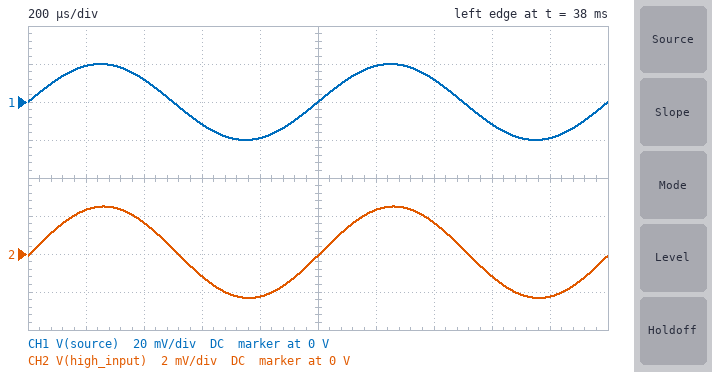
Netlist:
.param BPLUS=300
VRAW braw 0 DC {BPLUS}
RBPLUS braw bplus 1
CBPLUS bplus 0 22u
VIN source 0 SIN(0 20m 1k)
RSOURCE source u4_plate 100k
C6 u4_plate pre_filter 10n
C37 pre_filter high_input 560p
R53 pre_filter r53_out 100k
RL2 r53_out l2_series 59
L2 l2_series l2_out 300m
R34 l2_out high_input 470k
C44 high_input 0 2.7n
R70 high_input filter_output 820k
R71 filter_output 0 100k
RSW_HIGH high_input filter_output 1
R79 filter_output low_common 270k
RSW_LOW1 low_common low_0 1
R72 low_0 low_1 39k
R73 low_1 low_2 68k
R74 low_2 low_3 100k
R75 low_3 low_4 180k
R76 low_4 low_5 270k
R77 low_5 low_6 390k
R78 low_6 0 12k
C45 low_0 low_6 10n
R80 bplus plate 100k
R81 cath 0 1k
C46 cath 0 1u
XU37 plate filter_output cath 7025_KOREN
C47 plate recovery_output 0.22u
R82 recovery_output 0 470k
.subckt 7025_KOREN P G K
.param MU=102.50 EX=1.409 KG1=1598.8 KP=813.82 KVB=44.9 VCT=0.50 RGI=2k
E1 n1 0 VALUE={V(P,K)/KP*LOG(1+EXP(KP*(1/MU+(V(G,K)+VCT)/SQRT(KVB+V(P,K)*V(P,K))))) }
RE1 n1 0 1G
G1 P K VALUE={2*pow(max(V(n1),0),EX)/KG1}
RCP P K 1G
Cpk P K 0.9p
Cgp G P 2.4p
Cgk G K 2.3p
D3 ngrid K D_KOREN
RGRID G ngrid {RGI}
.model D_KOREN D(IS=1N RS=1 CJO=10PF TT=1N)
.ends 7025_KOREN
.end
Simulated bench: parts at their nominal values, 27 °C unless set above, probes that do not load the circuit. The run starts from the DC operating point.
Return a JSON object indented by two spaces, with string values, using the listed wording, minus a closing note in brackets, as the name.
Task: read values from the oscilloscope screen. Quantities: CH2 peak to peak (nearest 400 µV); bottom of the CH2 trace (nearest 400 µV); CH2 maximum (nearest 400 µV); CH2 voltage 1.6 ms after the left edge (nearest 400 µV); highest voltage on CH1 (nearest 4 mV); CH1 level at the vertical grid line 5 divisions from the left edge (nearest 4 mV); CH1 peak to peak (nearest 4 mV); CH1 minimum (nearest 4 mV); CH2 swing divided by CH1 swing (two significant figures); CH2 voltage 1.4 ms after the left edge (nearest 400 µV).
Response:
{
  "CH2 peak to peak": "4.8 mV",
  "bottom of the CH2 trace": "-2.4 mV",
  "CH2 maximum": "2.4 mV",
  "CH2 voltage 1.6 ms after the left edge": "-1.2 mV",
  "highest voltage on CH1": "20 mV",
  "CH1 level at the vertical grid line 5 divisions from the left edge": "0 V",
  "CH1 peak to peak": "40 mV",
  "CH1 minimum": "-20 mV",
  "CH2 swing divided by CH1 swing": "0.12",
  "CH2 voltage 1.4 ms after the left edge": "1.6 mV"
}
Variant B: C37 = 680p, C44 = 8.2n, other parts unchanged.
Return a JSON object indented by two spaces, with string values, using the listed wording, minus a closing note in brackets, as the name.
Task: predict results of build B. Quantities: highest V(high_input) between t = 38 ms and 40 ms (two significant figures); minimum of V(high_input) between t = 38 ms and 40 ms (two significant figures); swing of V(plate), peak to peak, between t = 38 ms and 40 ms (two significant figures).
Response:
{
  "highest V(high_input) between t = 38 ms and 40 ms": "1.3 mV",
  "minimum of V(high_input) between t = 38 ms and 40 ms": "-1.1 mV",
  "swing of V(plate), peak to peak, between t = 38 ms and 40 ms": "140 mV"
}
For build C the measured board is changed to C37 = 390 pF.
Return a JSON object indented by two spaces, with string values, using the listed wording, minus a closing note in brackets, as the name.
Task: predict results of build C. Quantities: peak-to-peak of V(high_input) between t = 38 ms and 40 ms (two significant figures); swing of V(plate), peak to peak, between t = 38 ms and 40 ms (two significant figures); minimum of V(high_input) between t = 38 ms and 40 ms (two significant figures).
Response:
{
  "peak-to-peak of V(high_input) between t = 38 ms and 40 ms": "3.9 mV",
  "swing of V(plate), peak to peak, between t = 38 ms and 40 ms": "230 mV",
  "minimum of V(high_input) between t = 38 ms and 40 ms": "-1.9 mV"
}
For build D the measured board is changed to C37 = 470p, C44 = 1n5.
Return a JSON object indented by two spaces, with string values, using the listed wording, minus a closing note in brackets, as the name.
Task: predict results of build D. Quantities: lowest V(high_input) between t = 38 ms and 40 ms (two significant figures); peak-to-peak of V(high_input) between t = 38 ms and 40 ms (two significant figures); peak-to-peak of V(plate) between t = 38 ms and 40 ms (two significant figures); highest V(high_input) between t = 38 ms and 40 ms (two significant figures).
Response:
{
  "lowest V(high_input) between t = 38 ms and 40 ms": "-2.7 mV",
  "peak-to-peak of V(high_input) between t = 38 ms and 40 ms": "5.5 mV",
  "peak-to-peak of V(plate) between t = 38 ms and 40 ms": "320 mV",
  "highest V(high_input) between t = 38 ms and 40 ms": "2.9 mV"
}
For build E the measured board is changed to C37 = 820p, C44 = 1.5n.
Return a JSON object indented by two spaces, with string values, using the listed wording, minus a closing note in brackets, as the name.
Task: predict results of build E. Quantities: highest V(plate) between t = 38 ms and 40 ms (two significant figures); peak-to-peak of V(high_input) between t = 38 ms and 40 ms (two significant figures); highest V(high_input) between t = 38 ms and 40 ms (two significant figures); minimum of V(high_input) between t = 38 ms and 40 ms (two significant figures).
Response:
{
  "highest V(plate) between t = 38 ms and 40 ms": "180 V",
  "peak-to-peak of V(high_input) between t = 38 ms and 40 ms": "7.7 mV",
  "highest V(high_input) between t = 38 ms and 40 ms": "3.9 mV",
  "minimum of V(high_input) between t = 38 ms and 40 ms": "-3.7 mV"
}
